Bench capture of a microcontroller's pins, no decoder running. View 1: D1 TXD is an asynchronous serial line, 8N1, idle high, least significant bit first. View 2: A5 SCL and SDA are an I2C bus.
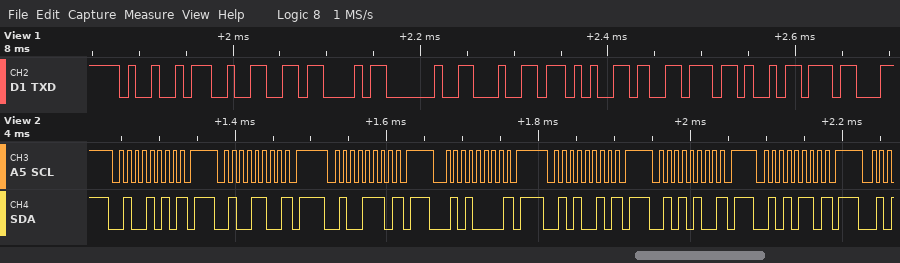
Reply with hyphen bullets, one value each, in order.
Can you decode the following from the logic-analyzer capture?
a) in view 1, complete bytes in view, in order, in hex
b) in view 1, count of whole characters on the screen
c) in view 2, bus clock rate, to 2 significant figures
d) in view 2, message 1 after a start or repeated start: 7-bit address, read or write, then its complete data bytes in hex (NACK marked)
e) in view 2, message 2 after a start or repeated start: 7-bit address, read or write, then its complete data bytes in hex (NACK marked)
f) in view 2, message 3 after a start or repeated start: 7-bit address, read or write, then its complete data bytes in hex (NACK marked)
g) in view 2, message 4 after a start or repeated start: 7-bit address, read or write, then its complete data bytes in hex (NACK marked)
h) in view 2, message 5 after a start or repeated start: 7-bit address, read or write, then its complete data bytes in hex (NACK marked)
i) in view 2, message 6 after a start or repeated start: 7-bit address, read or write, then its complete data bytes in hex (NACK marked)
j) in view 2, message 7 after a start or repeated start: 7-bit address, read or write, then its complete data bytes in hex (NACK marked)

- 0x49 0x32 0x43 0x20 0x64 0x65 0x76 0x69
- 8
- 100 kHz
- 0x25 write NACK
- 0x26 write NACK
- 0x27 write NACK
- 0x28 write NACK
- 0x29 write NACK
- 0x2A write NACK
- 0x2B write NACK
